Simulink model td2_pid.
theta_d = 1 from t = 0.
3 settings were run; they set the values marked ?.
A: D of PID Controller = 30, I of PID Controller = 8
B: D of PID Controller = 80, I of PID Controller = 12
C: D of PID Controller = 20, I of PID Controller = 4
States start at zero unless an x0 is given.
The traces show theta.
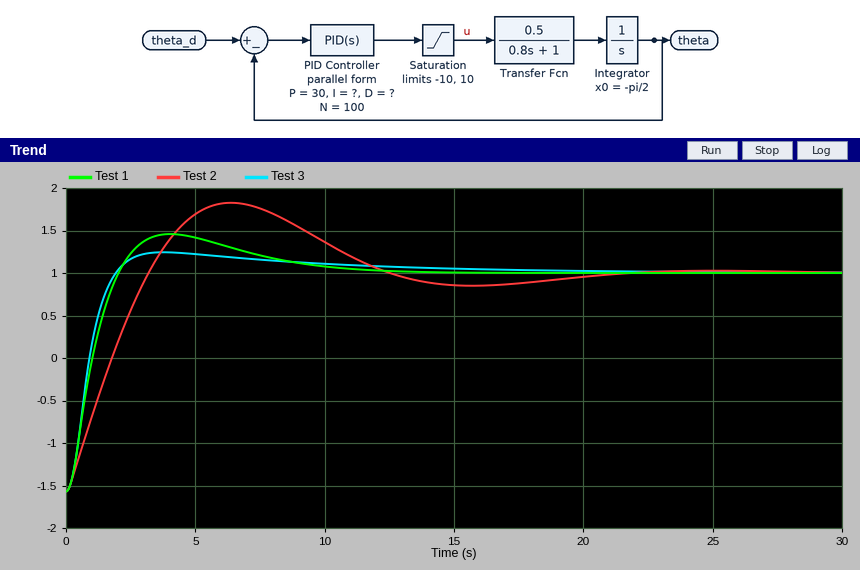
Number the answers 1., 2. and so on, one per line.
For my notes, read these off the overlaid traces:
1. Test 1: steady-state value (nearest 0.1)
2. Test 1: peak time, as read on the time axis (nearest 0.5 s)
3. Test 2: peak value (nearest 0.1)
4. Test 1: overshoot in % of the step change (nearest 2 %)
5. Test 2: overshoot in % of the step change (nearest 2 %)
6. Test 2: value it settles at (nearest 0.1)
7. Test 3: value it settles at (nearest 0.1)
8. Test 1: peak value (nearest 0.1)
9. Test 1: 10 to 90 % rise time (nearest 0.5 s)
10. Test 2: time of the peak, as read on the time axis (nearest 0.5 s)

1. 1.0
2. 4.0 s
3. 1.8
4. 18 %
5. 32 %
6. 1.0
7. 1.0
8. 1.5
9. 1.5 s
10. 6.5 s
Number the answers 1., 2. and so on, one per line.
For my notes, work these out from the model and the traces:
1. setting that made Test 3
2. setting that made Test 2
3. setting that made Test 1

1. C
2. B
3. A
